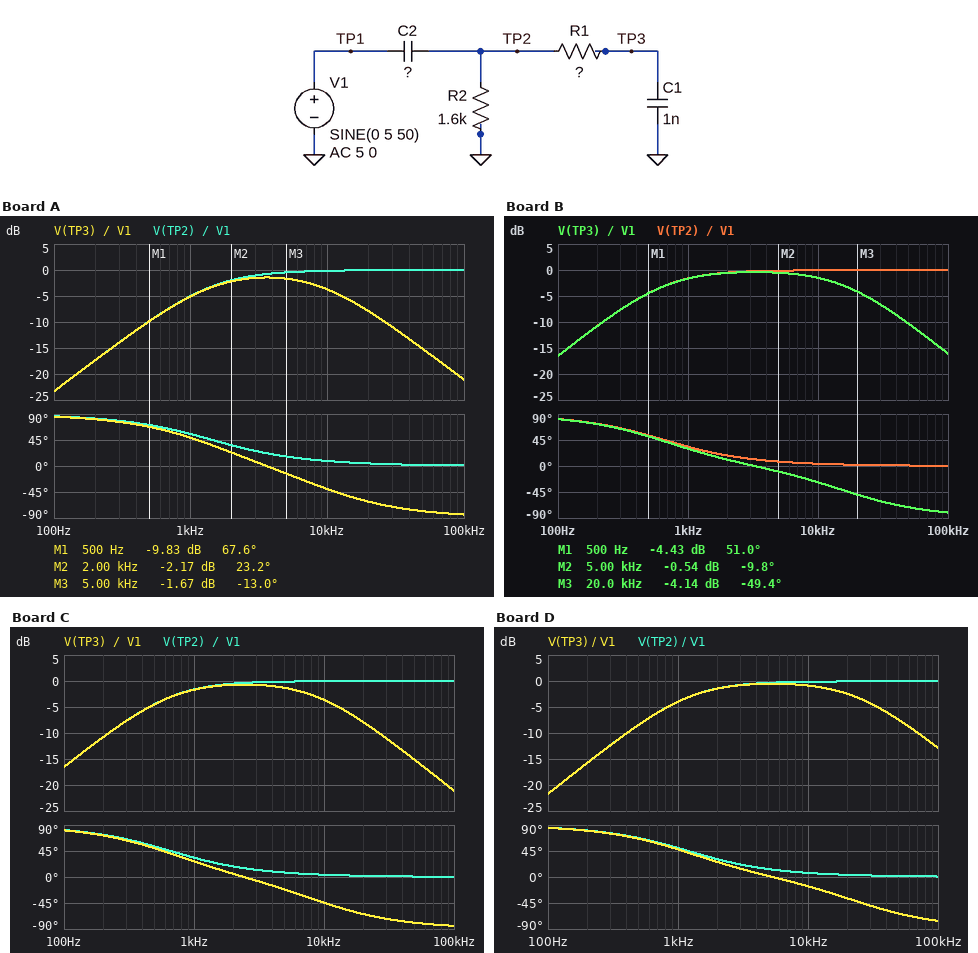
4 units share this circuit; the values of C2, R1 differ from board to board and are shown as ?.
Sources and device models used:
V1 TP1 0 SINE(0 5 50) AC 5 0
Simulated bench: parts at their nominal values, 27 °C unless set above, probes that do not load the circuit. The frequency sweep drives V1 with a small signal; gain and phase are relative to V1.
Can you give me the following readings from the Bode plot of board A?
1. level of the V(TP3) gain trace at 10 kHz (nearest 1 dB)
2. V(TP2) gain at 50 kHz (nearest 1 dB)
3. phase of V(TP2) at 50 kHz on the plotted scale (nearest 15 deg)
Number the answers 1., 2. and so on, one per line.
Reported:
1. -4 dB
2. 0 dB
3. 0 deg
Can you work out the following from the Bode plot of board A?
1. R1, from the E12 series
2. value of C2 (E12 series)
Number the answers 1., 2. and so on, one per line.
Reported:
1. 18 kΩ
2. 68 nF
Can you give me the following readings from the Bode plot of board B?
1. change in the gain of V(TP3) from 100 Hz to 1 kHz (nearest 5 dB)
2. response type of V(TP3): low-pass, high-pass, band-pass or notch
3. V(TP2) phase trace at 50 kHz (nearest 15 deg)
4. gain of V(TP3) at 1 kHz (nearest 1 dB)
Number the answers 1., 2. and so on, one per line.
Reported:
1. 15 dB
2. band-pass
3. 0 deg
4. -2 dB
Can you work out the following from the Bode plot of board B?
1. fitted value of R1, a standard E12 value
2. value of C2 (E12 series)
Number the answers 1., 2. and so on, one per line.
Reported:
1. 10 kΩ
2. 150 nF
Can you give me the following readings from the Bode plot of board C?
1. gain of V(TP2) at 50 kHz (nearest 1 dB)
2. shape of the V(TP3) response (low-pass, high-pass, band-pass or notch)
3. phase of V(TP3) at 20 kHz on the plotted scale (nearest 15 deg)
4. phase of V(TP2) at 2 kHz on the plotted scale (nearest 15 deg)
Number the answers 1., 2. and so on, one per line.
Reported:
1. 0 dB
2. band-pass
3. -60 deg
4. 15 deg
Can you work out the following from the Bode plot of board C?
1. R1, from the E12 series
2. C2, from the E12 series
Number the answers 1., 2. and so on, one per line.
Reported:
1. 18 kΩ
2. 150 nF
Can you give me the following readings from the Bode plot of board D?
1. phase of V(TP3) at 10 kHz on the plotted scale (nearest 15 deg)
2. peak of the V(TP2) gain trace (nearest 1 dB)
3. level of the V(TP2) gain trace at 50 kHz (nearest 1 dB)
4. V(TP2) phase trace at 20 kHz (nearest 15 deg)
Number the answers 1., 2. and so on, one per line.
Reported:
1. -15 deg
2. 0 dB
3. 0 dB
4. 0 deg
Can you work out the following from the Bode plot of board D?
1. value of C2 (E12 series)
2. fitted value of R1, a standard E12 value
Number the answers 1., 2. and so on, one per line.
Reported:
1. 82 nF
2. 6.8 kΩ
